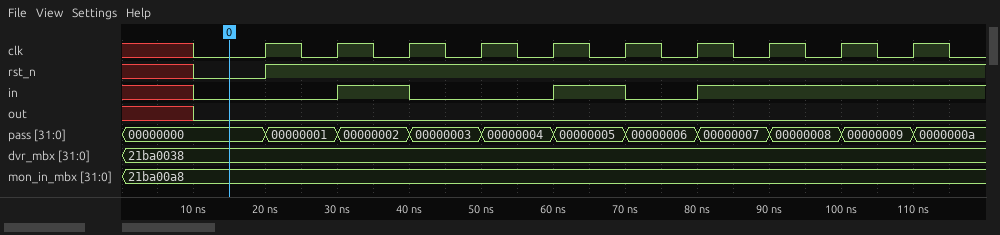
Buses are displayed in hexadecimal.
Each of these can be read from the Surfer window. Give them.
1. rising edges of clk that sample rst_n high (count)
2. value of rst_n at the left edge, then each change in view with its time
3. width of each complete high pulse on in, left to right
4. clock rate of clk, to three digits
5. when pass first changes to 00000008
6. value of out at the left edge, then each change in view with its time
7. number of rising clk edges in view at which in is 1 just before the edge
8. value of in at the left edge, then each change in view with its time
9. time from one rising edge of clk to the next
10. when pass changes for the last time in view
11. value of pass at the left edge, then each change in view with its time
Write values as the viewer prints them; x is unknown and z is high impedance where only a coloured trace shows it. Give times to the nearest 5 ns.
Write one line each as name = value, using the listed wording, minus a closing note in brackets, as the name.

rising edges of clk that sample rst_n high = 9
value of rst_n at the left edge, then each change in view with its time = x, 0 at 10 ns, 1 at 20 ns
width of each complete high pulse on in, left to right = 10 ns, 10 ns
clock rate of clk, to three digits = 100 MHz
when pass first changes to 00000008 = 90 ns
value of out at the left edge, then each change in view with its time = x, 0 at 10 ns
number of rising clk edges in view at which in is 1 just before the edge = 5
value of in at the left edge, then each change in view with its time = x, 0 at 10 ns, 1 at 30 ns, 0 at 40 ns, 1 at 60 ns, 0 at 70 ns, 1 at 80 ns
time from one rising edge of clk to the next = 10 ns
when pass changes for the last time in view = 110 ns
value of pass at the left edge, then each change in view with its time = 00000000, 00000001 at 20 ns, 00000002 at 30 ns, 00000003 at 40 ns, 00000004 at 50 ns, 00000005 at 60 ns, 00000006 at 70 ns, 00000007 at 80 ns, 00000008 at 90 ns, 00000009 at 100 ns, 0000000a at 110 ns
